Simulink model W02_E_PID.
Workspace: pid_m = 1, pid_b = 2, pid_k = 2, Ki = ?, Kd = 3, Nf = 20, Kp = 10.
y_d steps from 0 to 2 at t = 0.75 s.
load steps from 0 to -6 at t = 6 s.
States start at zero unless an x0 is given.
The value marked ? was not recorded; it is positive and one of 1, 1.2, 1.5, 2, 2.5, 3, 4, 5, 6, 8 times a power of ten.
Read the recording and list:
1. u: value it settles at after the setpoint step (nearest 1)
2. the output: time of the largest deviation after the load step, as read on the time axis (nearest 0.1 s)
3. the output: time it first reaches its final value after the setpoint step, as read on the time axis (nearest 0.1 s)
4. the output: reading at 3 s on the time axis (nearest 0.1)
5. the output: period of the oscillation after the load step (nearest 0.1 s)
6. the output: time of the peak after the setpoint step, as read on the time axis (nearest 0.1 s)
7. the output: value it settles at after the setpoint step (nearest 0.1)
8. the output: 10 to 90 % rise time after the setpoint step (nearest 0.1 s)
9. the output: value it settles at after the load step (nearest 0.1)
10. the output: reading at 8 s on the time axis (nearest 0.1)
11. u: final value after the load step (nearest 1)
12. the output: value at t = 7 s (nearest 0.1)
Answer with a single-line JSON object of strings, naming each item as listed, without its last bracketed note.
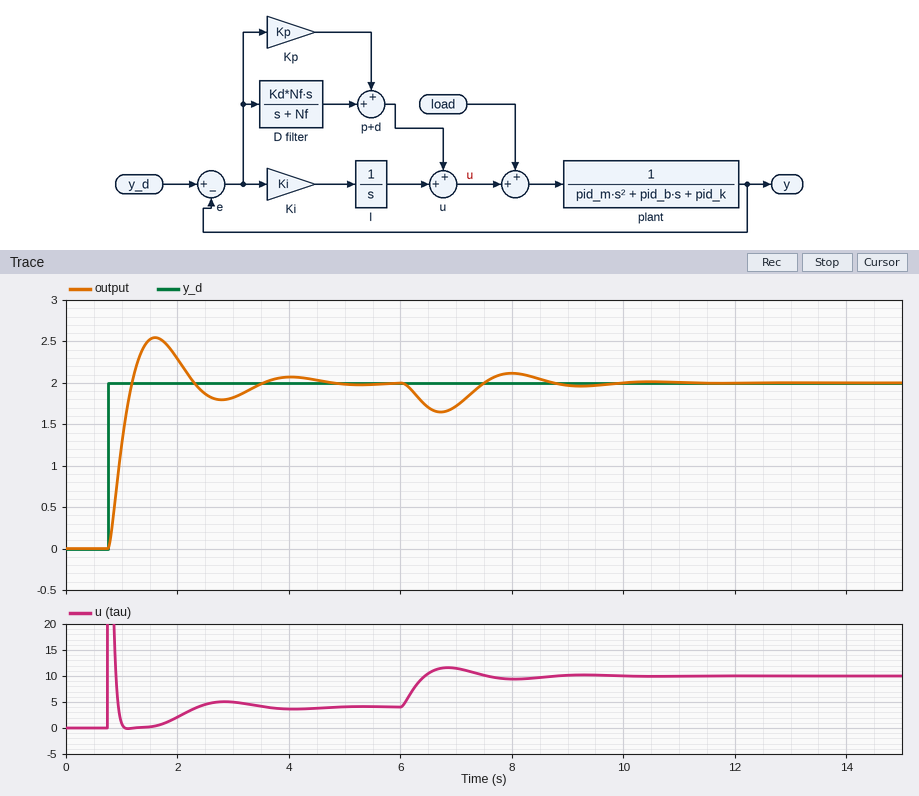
{"u: value it settles at after the setpoint step": "4", "the output: time of the largest deviation after the load step, as read on the time axis": "6.7 s", "the output: time it first reaches its final value after the setpoint step, as read on the time axis": "1.2 s", "the output: reading at 3 s on the time axis": "1.8", "the output: period of the oscillation after the load step": "2.5 s", "the output: time of the peak after the setpoint step, as read on the time axis": "1.6 s", "the output: value it settles at after the setpoint step": "2.0", "the output: 10 to 90 % rise time after the setpoint step": "0.3 s", "the output: value it settles at after the load step": "2.0", "the output: reading at 8 s on the time axis": "2.1", "u: final value after the load step": "10", "the output: value at t = 7 s": "1.7"}
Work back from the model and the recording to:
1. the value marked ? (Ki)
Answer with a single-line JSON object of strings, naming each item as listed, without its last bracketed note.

{"the value marked ?": "25"}
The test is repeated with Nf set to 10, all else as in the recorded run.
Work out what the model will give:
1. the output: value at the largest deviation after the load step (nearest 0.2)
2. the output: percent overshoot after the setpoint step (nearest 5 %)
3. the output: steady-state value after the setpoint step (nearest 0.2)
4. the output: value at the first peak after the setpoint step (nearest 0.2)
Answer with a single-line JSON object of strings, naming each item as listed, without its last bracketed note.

{"the output: value at the largest deviation after the load step": "1.6", "the output: percent overshoot after the setpoint step": "30 %", "the output: steady-state value after the setpoint step": "2.0", "the output: value at the first peak after the setpoint step": "2.6"}
